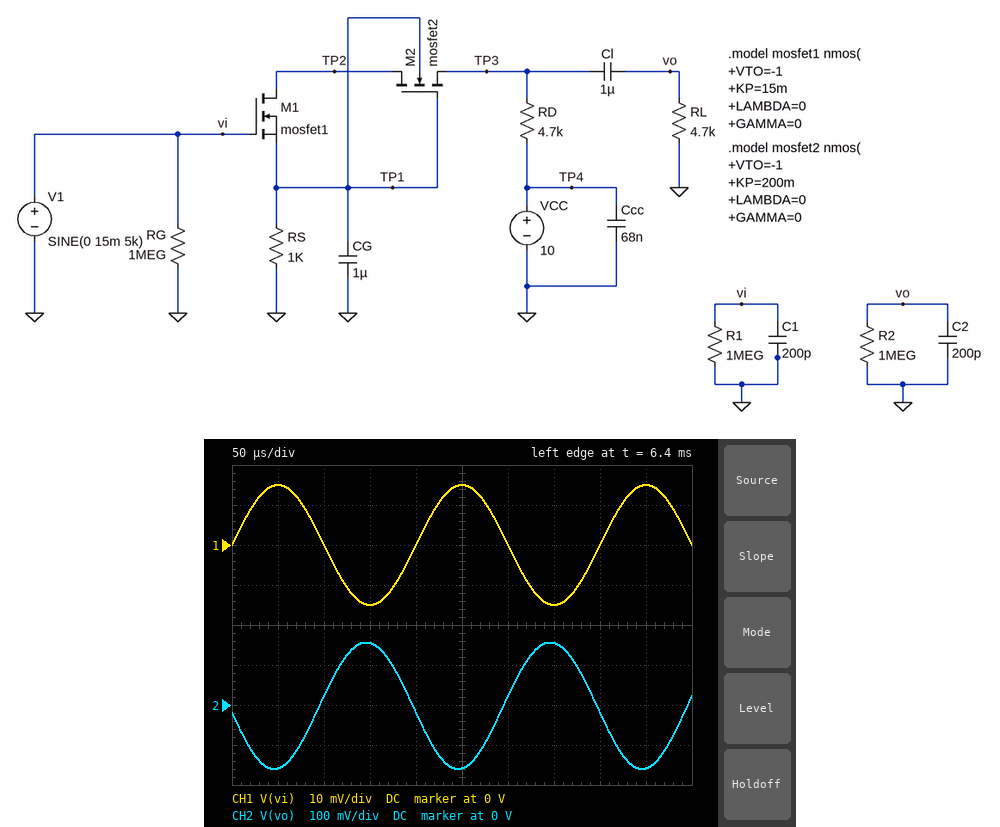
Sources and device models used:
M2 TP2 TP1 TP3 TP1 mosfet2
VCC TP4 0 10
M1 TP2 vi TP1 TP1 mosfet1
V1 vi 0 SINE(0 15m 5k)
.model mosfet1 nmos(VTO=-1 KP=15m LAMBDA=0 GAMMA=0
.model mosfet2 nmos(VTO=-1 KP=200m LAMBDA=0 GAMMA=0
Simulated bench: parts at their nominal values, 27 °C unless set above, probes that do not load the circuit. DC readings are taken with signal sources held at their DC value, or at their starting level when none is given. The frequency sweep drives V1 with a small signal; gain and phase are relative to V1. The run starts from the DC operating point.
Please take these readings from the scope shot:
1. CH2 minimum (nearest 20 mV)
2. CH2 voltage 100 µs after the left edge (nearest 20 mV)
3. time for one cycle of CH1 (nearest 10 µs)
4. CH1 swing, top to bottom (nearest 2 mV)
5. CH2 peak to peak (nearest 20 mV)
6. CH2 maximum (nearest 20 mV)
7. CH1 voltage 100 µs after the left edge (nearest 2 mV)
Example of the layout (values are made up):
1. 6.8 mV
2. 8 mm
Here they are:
1. -160 mV
2. 20 mV
3. 200 µs
4. 30 mV
5. 320 mV
6. 160 mV
7. 0 V
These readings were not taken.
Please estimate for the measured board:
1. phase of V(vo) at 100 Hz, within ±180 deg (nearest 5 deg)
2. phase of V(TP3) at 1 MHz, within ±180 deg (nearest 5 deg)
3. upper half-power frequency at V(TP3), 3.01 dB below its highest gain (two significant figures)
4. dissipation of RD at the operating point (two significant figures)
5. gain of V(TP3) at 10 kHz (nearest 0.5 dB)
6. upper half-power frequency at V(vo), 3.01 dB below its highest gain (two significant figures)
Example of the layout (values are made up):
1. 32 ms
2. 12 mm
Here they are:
1. -145 deg
2. 110 deg
3. 340 kHz
4. 2.3 mW
5. 20.5 dB
6. 340 kHz
